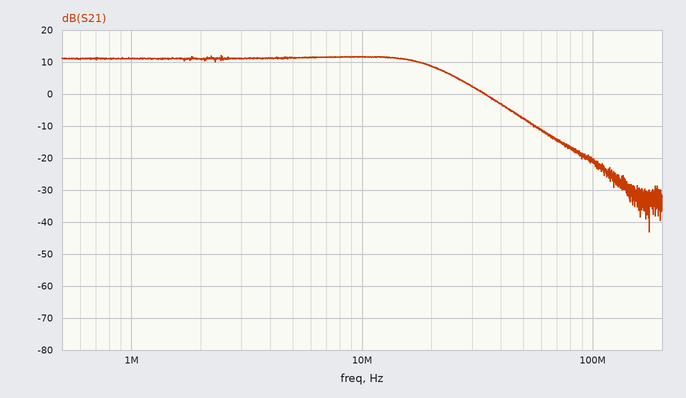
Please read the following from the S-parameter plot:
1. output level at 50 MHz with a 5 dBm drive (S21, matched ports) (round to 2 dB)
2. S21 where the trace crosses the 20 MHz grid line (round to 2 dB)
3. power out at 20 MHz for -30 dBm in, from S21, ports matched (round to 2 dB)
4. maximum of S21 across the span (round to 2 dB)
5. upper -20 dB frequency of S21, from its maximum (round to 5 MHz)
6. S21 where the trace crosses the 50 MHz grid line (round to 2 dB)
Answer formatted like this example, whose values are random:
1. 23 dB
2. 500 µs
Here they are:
1. -2 dBm
2. 8 dB
3. -22 dBm
4. 12 dB
5. 50 MHz
6. -8 dB
